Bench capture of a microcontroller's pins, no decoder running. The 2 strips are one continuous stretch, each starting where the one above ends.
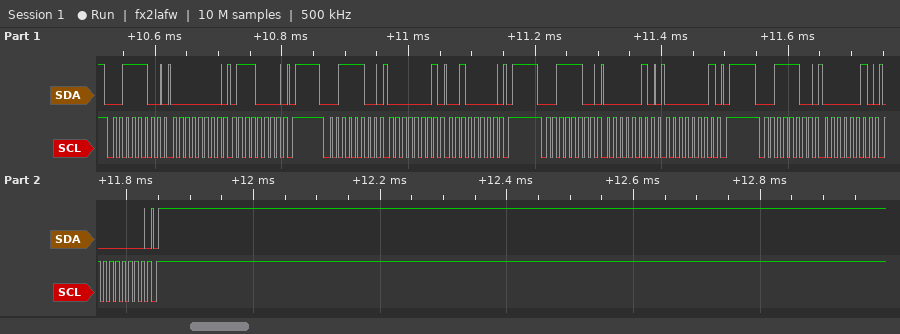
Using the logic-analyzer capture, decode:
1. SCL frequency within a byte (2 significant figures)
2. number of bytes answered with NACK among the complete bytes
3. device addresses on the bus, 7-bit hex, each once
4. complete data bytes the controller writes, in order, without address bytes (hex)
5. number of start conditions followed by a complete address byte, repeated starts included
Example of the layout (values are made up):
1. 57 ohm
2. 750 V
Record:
1. 100 kHz
2. 0
3. 0x1E
4. 00 70 01 20 02 01 02 00
5. 4
